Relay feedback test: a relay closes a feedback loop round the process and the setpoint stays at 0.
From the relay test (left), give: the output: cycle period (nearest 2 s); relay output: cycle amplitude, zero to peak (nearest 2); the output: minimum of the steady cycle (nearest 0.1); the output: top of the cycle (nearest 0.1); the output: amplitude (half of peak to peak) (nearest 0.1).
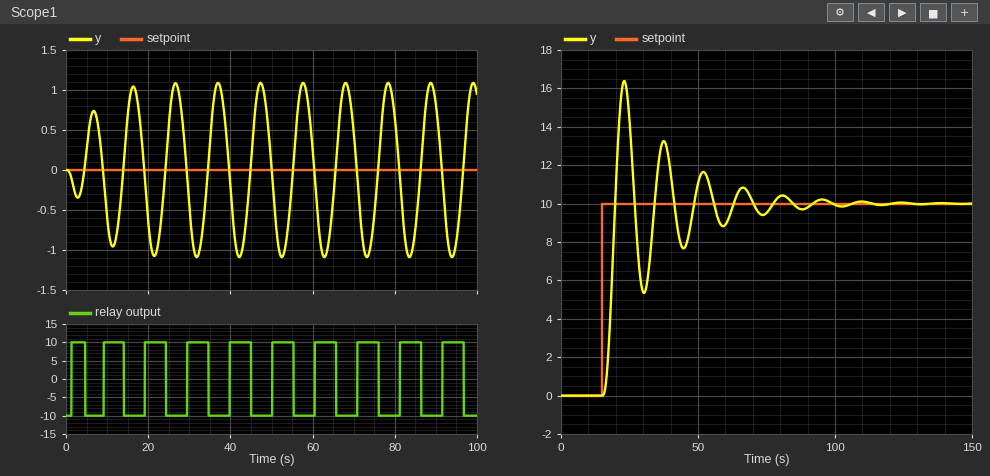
10 s
10
-1.1
1.1
1.1
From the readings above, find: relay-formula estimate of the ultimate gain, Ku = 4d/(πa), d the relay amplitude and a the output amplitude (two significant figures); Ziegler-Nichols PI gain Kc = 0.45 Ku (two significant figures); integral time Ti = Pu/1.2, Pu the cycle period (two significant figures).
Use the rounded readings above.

12
5.4
8.3 s
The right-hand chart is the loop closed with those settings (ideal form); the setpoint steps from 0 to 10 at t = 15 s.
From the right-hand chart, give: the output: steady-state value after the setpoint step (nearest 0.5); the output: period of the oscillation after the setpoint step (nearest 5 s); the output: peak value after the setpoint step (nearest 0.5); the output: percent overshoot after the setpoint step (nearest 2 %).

10.0
15 s
16.5
64 %
